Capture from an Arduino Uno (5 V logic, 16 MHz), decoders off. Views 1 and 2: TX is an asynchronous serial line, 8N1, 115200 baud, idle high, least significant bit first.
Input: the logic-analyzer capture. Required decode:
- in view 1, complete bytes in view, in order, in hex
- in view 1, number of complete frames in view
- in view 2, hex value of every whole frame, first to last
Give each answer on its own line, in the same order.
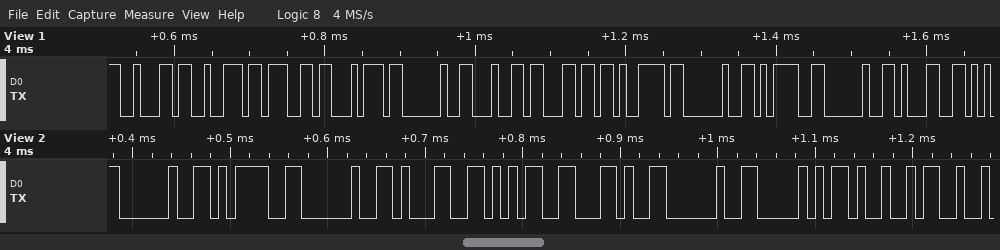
62 72 67 74 20 64 6C 79 20 3D 20 31
12
0x20 0x3D 0x20 0x31 0x35 0x2C 0x20 0x50 0x49
